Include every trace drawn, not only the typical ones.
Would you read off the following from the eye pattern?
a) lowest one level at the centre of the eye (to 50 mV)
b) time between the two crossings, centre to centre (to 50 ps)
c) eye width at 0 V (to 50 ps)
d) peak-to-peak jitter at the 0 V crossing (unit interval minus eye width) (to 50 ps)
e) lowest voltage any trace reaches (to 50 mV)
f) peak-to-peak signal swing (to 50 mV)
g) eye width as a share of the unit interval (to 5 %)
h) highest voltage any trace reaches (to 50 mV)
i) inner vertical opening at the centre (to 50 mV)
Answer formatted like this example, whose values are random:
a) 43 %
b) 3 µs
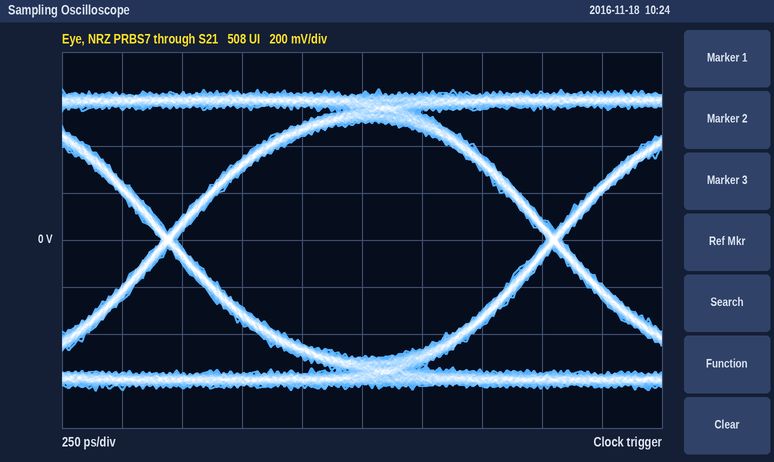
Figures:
a) 500 mV
b) 1.60 ns
c) 1.55 ns
d) 50 ps
e) -650 mV
f) 1.30 V
g) 95 %
h) 650 mV
i) 1.00 V
